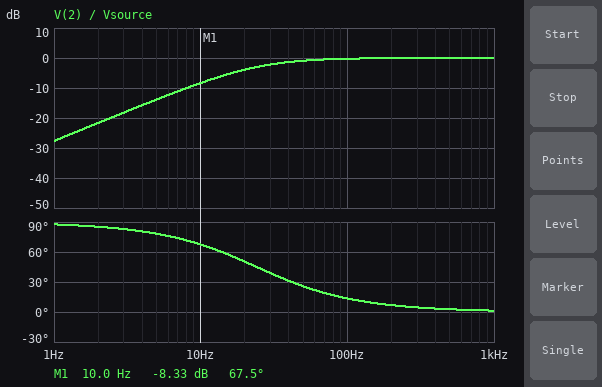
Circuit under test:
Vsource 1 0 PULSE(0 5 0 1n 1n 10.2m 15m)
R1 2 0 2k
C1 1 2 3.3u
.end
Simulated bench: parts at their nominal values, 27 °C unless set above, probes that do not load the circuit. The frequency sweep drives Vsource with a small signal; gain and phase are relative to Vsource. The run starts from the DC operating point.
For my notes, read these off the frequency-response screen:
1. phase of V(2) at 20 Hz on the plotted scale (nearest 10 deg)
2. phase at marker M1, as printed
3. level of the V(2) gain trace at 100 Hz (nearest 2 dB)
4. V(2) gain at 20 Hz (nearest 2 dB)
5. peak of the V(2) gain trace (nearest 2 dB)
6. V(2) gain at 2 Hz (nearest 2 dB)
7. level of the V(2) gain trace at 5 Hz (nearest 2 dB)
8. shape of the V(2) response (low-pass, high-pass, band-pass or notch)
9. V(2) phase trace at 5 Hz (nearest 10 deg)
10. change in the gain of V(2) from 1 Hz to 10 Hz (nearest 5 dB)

50 deg
67.5 deg
0 dB
-4 dB
0 dB
-22 dB
-14 dB
high-pass
80 deg
20 dB
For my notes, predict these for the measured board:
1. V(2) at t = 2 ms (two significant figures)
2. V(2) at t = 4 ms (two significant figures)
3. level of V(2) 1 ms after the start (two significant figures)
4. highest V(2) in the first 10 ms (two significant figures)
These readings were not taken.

3.7 V
2.7 V
4.3 V
5.0 V
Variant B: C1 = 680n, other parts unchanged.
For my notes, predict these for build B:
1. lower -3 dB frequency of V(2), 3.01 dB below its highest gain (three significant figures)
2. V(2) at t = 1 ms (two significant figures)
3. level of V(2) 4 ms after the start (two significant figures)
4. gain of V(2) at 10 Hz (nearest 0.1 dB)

117 Hz
2.4 V
260 mV
-21.4 dB
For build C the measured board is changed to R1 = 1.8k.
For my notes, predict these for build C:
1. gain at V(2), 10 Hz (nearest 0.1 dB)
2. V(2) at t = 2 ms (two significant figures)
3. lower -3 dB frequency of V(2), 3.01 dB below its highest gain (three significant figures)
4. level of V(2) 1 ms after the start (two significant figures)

-9.1 dB
3.6 V
26.8 Hz
4.2 V
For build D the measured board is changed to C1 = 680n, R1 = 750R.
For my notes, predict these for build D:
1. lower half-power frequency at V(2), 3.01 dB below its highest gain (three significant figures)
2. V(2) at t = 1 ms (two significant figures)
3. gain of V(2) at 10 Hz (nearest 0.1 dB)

312 Hz
700 mV
-29.9 dB
